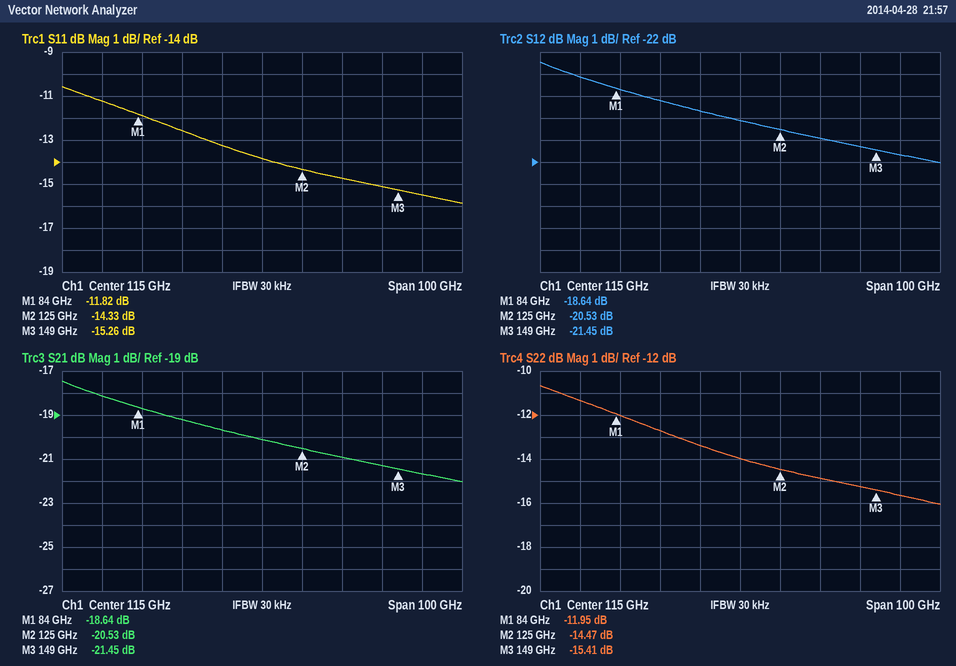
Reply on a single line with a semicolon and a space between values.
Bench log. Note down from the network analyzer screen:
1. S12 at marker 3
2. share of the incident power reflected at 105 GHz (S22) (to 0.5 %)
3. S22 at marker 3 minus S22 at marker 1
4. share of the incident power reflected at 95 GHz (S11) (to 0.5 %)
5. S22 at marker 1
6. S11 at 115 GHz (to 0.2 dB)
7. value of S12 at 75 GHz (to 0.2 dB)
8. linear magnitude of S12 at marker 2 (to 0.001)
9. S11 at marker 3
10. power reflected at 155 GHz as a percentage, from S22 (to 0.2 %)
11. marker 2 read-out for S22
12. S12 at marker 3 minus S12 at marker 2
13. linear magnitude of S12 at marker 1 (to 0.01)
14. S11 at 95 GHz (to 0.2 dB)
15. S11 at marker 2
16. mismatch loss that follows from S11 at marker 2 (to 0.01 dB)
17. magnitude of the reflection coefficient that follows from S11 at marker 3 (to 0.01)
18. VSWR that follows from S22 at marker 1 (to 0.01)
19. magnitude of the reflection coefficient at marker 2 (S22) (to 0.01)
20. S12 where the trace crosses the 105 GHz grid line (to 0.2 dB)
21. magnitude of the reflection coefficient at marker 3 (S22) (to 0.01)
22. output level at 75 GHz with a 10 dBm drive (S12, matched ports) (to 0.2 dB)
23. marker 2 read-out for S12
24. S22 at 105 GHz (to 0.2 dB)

-21.45 dB; 4.5 %; -3.46 dB; 5.5 %; -11.95 dB; -13.8 dB; -18.2 dB; 0.094; -15.26 dB; 2.8 %; -14.47 dB; -0.92 dB; 0.12; -12.6 dB; -14.33 dB; 0.16 dB; 0.17; 1.68; 0.19; -19.6 dB; 0.17; -8.2 dBm; -20.53 dB; -13.4 dB
